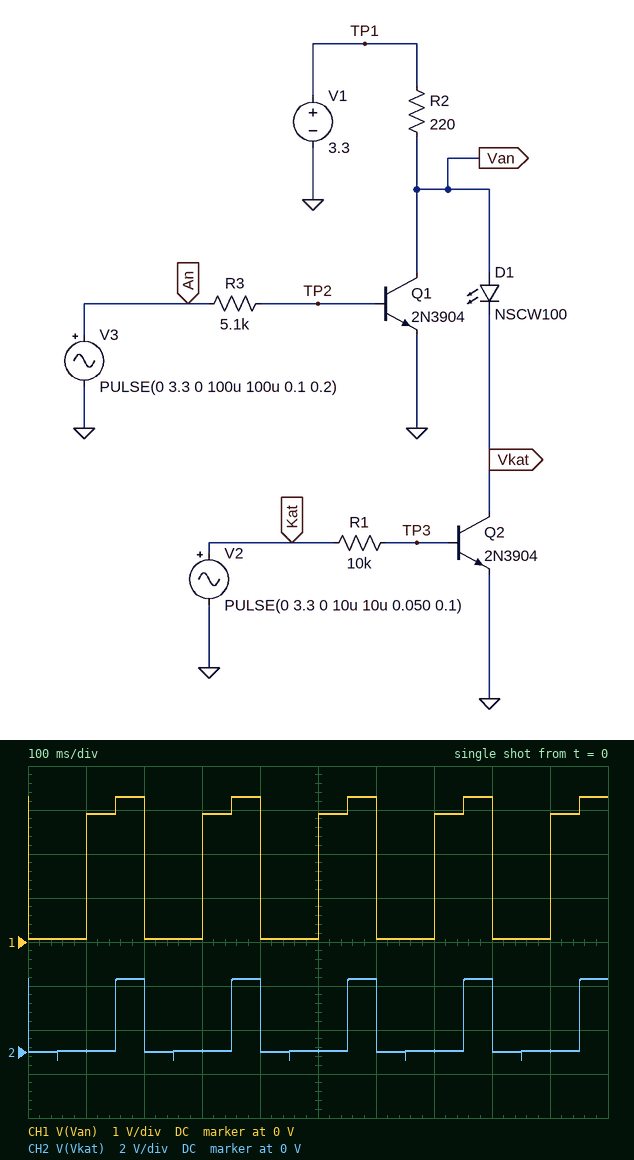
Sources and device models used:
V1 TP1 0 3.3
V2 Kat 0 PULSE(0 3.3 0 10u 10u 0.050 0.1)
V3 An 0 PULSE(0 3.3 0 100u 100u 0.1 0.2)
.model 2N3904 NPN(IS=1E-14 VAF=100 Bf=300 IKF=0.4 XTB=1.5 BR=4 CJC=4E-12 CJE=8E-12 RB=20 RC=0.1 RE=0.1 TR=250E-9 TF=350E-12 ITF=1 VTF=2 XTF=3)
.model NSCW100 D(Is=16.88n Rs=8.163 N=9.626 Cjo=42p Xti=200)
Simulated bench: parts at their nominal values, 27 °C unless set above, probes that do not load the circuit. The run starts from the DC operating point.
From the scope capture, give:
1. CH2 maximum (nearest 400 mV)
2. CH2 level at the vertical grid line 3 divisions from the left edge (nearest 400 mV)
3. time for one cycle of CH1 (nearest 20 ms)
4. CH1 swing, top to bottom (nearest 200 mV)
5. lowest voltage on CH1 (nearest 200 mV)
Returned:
3.2 V
0 V
200 ms
3.2 V
0 V
